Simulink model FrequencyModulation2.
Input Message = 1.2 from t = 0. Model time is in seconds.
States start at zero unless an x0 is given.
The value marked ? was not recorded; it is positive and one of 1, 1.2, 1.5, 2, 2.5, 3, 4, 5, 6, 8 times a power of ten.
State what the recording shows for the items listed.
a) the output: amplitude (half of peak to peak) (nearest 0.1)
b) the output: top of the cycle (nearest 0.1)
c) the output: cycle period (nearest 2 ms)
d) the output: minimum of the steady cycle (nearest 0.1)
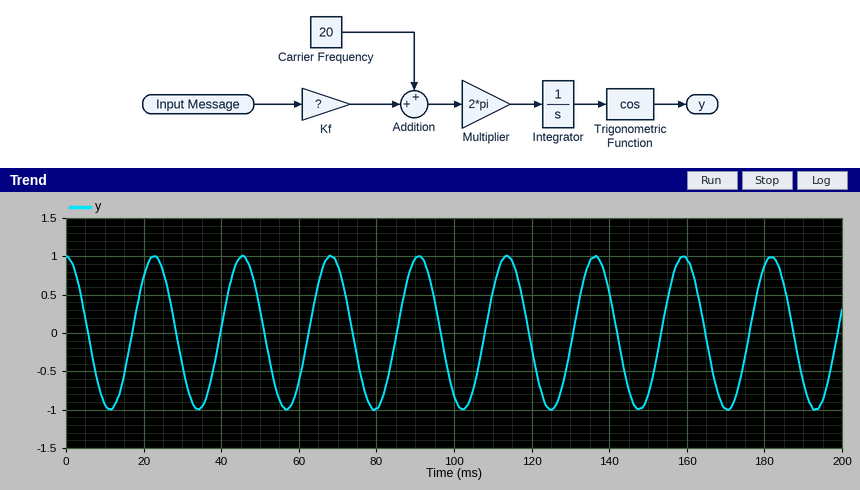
1.0
1.0
22 ms
-1.0
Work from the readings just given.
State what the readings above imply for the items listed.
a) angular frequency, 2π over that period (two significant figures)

0.29 rad/ms
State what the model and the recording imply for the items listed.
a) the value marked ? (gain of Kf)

20
